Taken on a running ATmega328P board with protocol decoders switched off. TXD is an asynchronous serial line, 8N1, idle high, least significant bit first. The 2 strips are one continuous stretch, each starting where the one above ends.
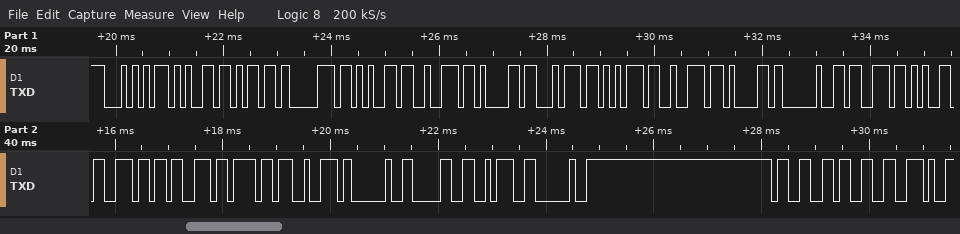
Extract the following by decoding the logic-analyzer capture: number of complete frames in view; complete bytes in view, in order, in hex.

25
0x54 0x65 0x6D 0x70 0x65 0x72 0x61 0x74 0x75 0x72 0x61 0x20 0x73 0x65 0x6E 0x73 0x6F 0x72 0x20 0x30 0x3A 0x20 0x33 0x33 0x2E
